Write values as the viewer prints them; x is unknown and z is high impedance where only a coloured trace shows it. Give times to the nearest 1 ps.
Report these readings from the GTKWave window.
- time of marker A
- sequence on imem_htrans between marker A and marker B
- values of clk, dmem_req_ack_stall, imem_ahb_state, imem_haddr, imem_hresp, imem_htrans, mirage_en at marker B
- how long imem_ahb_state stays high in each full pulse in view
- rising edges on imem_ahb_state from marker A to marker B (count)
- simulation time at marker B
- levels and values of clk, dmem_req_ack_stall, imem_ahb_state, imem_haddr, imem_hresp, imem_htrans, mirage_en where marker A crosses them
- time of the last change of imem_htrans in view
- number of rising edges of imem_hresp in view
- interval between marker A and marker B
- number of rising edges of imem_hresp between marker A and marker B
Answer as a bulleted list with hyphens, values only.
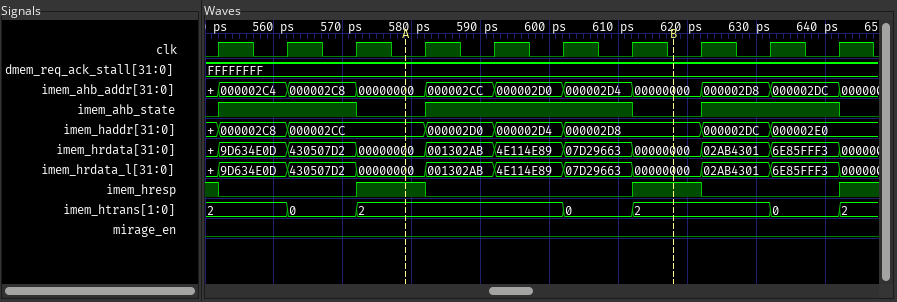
- 579 ps
- 2, 0, 2
- clk=0, dmem_req_ack_stall=FFFFFFFF, imem_ahb_state=0, imem_haddr=000002D8, imem_hresp=1, imem_htrans=2, mirage_en=0
- 20 ps, 30 ps, 20 ps
- 1
- 618 ps
- clk=0, dmem_req_ack_stall=FFFFFFFF, imem_ahb_state=0, imem_haddr=000002CC, imem_hresp=1, imem_htrans=2, mirage_en=0
- 642 ps
- 3
- 39 ps
- 1
